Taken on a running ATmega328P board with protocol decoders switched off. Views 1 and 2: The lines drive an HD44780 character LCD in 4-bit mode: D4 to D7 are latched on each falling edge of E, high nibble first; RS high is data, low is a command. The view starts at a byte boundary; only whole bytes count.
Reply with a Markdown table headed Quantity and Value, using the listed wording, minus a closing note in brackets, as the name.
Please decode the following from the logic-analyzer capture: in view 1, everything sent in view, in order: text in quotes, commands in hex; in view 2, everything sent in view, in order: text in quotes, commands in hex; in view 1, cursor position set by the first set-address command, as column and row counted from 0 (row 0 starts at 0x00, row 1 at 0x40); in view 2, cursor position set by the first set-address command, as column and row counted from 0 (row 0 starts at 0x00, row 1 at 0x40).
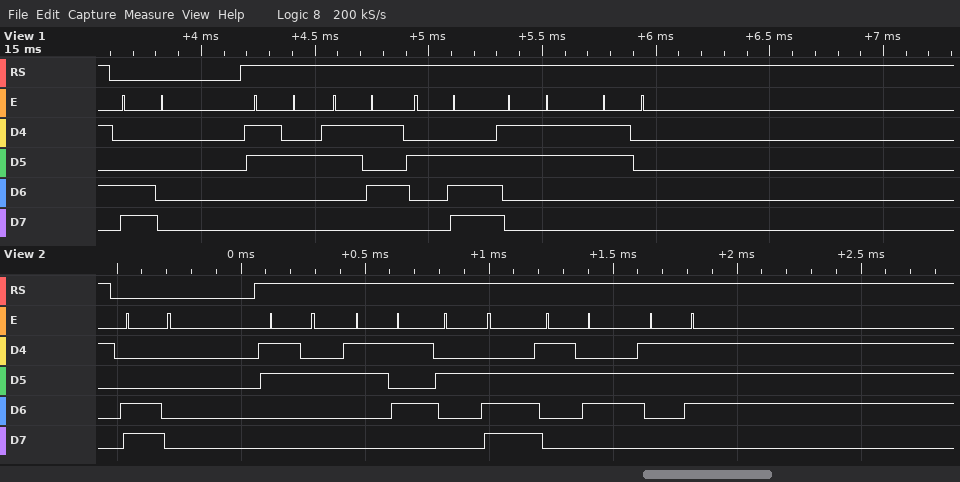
| Quantity | Value |
|---|---|
| in view 1, everything sent in view, in order: text in quotes, commands in hex | 0xC0 "25.30" |
| in view 2, everything sent in view, in order: text in quotes, commands in hex | 0xC0 "25.67" |
| in view 1, cursor position set by the first set-address command, as column and row counted from 0 | column 0, row 1 |
| in view 2, cursor position set by the first set-address command, as column and row counted from 0 | column 0, row 1 |
